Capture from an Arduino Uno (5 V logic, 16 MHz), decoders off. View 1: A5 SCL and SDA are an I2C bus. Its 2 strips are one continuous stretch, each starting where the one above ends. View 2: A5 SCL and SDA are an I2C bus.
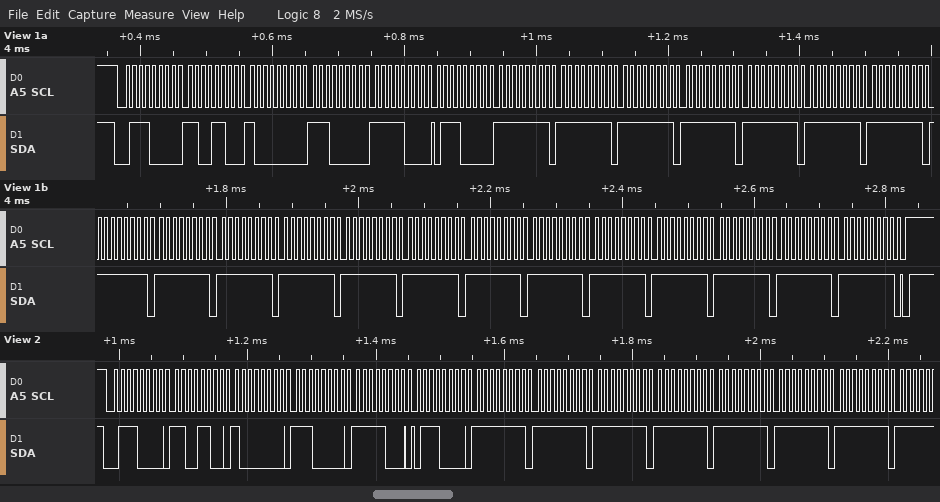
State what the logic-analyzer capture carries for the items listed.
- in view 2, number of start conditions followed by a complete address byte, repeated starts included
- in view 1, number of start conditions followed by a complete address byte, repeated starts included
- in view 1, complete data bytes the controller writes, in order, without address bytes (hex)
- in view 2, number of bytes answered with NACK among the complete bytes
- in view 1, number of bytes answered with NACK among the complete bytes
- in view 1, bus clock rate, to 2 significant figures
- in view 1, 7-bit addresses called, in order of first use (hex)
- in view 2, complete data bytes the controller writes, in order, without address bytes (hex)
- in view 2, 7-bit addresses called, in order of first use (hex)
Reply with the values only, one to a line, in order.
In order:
1
1
CC 80 E0 F8 70 FF FF FF FF FF FF FF FF FF FF FF FF FF FF FF FF FF FF FF FF
0
0
100 kHz
0x38
CC 80 E0 F8 70 FF FF FF FF FF FF FF
0x38
